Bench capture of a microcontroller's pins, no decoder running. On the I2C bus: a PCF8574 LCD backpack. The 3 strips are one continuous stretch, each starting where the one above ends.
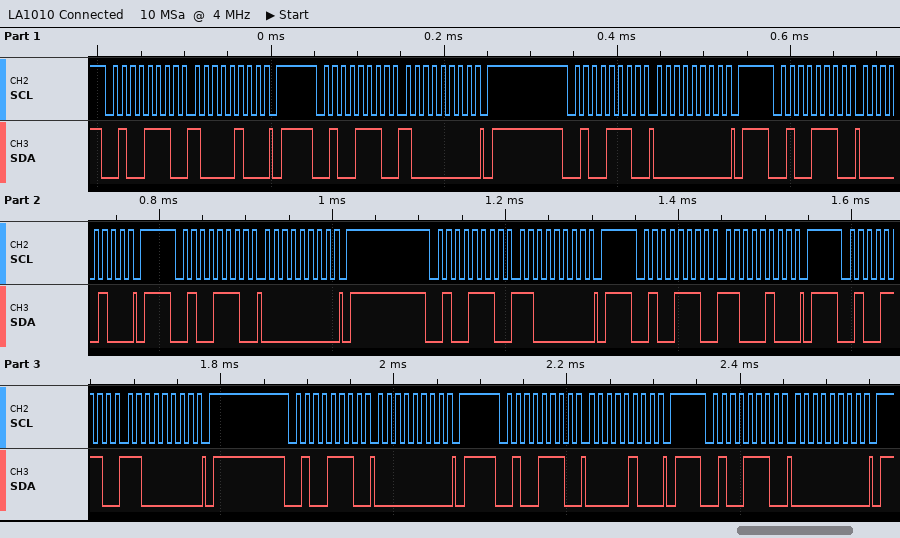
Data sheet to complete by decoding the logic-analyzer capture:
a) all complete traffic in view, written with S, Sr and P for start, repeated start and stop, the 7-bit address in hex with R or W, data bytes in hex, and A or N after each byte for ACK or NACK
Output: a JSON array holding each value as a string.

["S 27W A 84 A P S 27W A 80 A P S 27W A 00 A P S 27W A 04 A P S 27W A 00 A P S 27W A C0 A P S 27W A C4 A P S 27W A C0 A P S 27W A 00 A P S 27W A 04 A P S 27W A 00 A P"]
